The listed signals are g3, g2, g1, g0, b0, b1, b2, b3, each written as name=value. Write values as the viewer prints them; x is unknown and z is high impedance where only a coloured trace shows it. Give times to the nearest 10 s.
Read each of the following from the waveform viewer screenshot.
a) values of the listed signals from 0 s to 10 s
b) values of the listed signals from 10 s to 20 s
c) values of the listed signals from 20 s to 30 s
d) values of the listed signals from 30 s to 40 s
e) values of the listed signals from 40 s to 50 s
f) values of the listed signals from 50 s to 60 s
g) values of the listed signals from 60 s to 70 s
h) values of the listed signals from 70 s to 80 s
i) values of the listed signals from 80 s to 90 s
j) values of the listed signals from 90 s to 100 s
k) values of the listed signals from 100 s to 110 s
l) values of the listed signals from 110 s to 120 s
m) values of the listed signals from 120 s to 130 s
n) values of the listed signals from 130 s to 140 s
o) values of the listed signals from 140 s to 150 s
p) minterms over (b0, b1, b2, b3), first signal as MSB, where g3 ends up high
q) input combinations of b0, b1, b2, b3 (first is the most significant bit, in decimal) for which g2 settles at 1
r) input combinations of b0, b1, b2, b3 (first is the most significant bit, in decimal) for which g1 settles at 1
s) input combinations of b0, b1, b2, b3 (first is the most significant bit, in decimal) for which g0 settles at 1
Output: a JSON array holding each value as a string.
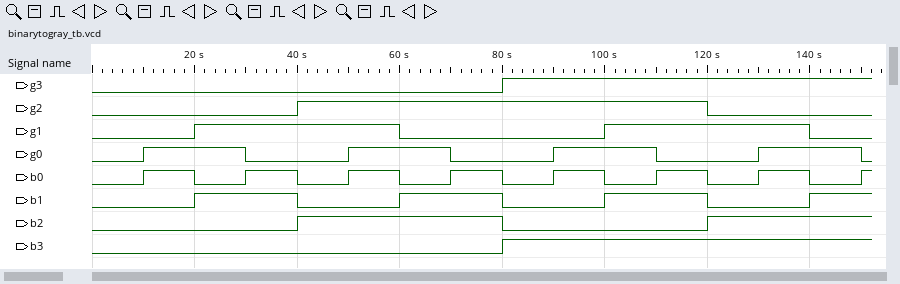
["g3=0, g2=0, g1=0, g0=0, b0=0, b1=0, b2=0, b3=0", "g3=0, g2=0, g1=0, g0=1, b0=1, b1=0, b2=0, b3=0", "g3=0, g2=0, g1=1, g0=1, b0=0, b1=1, b2=0, b3=0", "g3=0, g2=0, g1=1, g0=0, b0=1, b1=1, b2=0, b3=0", "g3=0, g2=1, g1=1, g0=0, b0=0, b1=0, b2=1, b3=0", "g3=0, g2=1, g1=1, g0=1, b0=1, b1=0, b2=1, b3=0", "g3=0, g2=1, g1=0, g0=1, b0=0, b1=1, b2=1, b3=0", "g3=0, g2=1, g1=0, g0=0, b0=1, b1=1, b2=1, b3=0", "g3=1, g2=1, g1=0, g0=0, b0=0, b1=0, b2=0, b3=1", "g3=1, g2=1, g1=0, g0=1, b0=1, b1=0, b2=0, b3=1", "g3=1, g2=1, g1=1, g0=1, b0=0, b1=1, b2=0, b3=1", "g3=1, g2=1, g1=1, g0=0, b0=1, b1=1, b2=0, b3=1", "g3=1, g2=0, g1=1, g0=0, b0=0, b1=0, b2=1, b3=1", "g3=1, g2=0, g1=1, g0=1, b0=1, b1=0, b2=1, b3=1", "g3=1, g2=0, g1=0, g0=1, b0=0, b1=1, b2=1, b3=1", "1, 3, 5, 7, 9, 11, 13, 15", "1, 2, 5, 6, 9, 10, 13, 14", "2, 3, 4, 5, 10, 11, 12, 13", "4, 5, 6, 7, 8, 9, 10, 11"]
